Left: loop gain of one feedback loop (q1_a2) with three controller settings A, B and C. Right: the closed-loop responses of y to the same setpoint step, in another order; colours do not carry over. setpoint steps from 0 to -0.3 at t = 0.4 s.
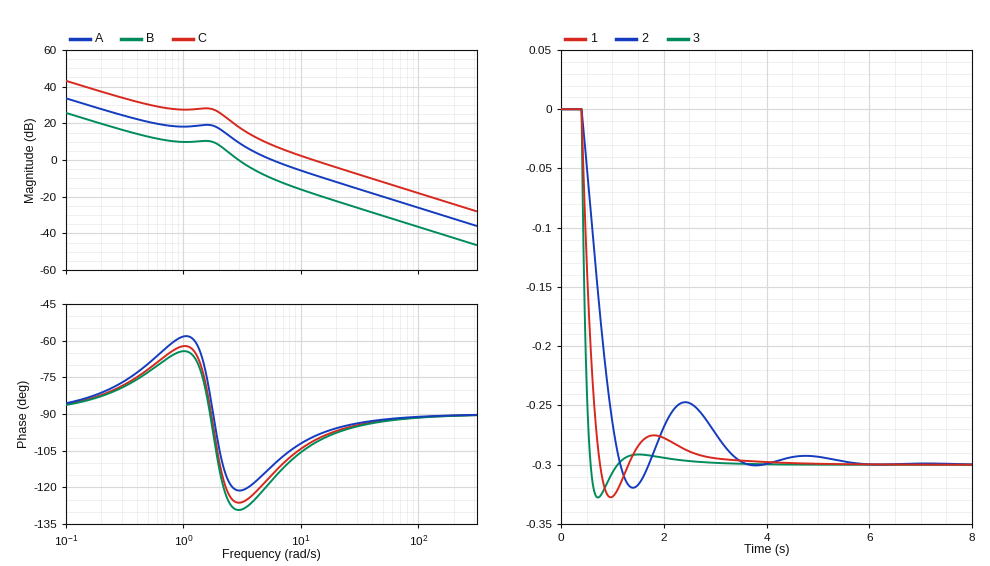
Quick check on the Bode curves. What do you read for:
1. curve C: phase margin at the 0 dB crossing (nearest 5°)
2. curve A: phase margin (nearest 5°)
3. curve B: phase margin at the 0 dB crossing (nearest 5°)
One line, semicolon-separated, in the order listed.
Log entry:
80°; 70°; 50°
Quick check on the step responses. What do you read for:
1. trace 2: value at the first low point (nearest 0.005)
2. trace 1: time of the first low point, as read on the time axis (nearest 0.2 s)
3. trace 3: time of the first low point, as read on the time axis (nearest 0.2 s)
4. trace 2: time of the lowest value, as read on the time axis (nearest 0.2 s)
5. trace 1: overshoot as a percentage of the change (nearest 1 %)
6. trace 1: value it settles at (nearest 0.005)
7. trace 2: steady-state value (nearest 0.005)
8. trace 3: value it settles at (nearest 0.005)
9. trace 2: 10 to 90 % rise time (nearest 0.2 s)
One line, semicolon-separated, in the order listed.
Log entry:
-0.320; 1.0 s; 0.8 s; 1.4 s; 9 %; -0.300; -0.300; -0.300; 0.6 s
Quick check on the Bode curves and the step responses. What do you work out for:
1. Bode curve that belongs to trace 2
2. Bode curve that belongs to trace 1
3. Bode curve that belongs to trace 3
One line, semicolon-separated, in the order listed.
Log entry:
B; A; C
